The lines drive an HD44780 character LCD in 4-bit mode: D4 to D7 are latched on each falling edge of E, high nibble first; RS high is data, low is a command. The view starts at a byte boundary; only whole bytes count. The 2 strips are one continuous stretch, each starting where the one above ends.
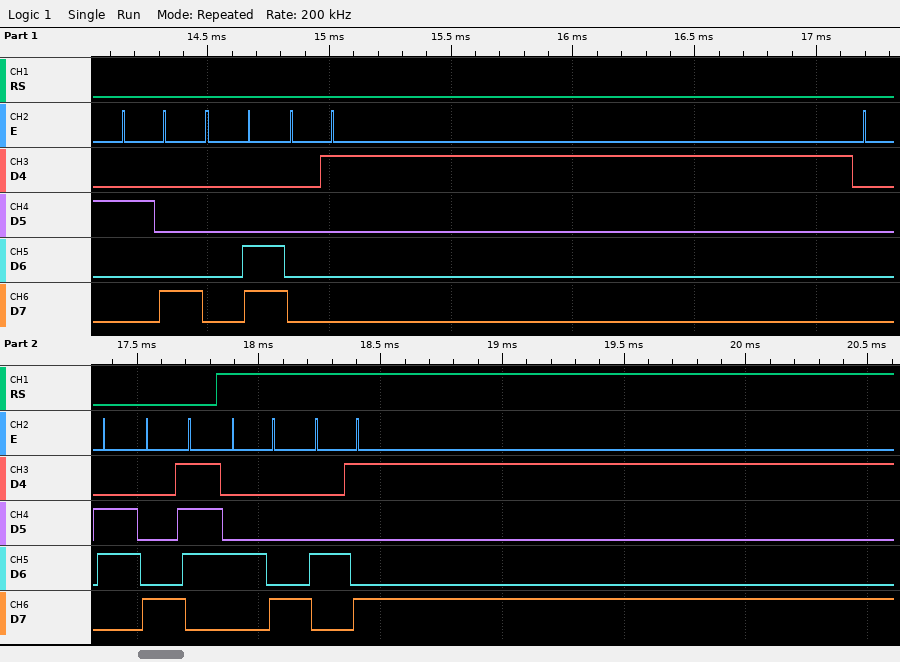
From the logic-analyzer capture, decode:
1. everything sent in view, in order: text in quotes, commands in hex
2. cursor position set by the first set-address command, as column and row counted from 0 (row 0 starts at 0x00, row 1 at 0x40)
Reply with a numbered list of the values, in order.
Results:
1. 0x28 0x0C 0x01 0x06 0x87 "HI"
2. column 7, row 0
